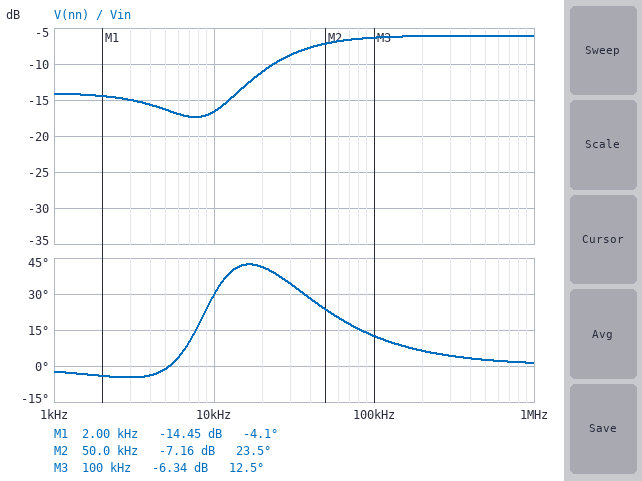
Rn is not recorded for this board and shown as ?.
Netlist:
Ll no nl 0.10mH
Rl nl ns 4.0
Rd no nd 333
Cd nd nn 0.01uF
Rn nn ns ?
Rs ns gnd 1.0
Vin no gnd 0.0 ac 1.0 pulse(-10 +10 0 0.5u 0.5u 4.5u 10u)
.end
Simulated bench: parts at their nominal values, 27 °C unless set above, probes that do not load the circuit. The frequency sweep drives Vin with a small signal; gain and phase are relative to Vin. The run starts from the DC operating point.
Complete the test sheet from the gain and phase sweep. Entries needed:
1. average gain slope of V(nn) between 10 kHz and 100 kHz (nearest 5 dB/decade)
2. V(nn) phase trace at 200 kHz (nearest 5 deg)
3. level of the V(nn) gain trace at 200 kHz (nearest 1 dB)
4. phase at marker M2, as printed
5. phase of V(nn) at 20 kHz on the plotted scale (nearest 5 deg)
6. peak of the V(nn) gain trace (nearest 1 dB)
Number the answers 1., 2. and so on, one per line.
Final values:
1. 10 dB/decade
2. 5 deg
3. -6 dB
4. 23.5 deg
5. 40 deg
6. -6 dB
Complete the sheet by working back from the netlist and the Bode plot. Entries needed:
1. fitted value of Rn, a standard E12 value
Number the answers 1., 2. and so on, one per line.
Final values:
1. 330 Ω
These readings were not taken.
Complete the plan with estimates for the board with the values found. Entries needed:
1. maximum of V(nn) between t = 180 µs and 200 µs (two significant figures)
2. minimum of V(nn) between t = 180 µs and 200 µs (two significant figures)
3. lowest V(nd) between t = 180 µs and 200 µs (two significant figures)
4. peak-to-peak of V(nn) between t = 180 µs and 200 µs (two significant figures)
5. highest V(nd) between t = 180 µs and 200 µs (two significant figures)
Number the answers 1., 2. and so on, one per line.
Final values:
1. 6.4 V
2. -6.4 V
3. -6.8 V
4. 13 V
5. 6.8 V
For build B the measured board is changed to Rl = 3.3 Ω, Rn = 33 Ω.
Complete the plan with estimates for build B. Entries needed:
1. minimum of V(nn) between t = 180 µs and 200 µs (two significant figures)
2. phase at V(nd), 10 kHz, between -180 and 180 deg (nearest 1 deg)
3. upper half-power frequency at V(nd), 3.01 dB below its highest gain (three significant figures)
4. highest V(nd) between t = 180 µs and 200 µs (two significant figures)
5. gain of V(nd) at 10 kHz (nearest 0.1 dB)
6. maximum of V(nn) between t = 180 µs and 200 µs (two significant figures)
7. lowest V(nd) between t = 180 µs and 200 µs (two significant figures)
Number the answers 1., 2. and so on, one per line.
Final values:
1. -1.2 V
2. -11 deg
3. 46.1 kHz
4. 6.2 V
5. 0 dB
6. 1.2 V
7. -6.2 V
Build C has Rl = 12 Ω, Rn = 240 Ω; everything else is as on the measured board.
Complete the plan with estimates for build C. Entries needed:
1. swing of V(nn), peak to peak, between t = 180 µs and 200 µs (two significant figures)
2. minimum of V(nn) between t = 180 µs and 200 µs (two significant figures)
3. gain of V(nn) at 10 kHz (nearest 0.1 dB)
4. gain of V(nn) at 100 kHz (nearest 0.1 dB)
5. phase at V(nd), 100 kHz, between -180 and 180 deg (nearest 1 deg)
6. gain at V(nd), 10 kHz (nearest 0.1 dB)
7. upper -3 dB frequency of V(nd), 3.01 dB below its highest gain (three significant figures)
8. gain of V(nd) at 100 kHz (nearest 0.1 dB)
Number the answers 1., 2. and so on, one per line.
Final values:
1. 11 V
2. -5.5 V
3. -17.0 dB
4. -7.9 dB
5. -19 deg
6. -0.4 dB
7. 36.7 kHz
8. -6.2 dB
